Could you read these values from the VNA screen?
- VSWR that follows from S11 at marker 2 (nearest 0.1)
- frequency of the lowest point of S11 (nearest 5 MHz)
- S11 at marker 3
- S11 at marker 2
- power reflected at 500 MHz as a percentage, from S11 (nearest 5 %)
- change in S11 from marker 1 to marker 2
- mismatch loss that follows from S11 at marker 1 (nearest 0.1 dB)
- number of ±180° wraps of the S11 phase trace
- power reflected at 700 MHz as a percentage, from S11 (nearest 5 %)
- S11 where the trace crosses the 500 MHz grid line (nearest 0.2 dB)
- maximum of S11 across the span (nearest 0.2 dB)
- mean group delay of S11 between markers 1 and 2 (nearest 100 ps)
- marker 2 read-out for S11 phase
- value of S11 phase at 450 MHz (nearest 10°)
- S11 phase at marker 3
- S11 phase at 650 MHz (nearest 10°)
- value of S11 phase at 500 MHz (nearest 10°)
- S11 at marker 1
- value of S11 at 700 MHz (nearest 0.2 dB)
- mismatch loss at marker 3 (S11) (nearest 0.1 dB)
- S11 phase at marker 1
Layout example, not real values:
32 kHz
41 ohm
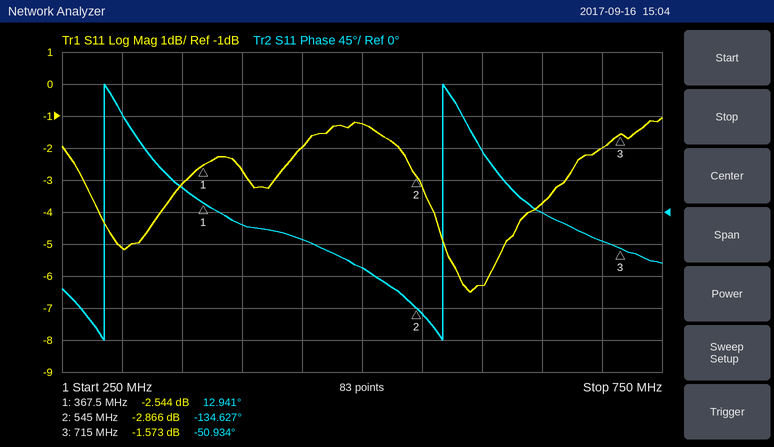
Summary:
6.1
590 MHz
-1.573 dB
-2.866 dB
75 %
-0.322 dB
3.5 dB
2
65 %
-1.2 dB
-1.0 dB
2.3 ns
-134.627°
-40°
-50.934°
0°
-80°
-2.544 dB
-2.0 dB
5.2 dB
12.941°
